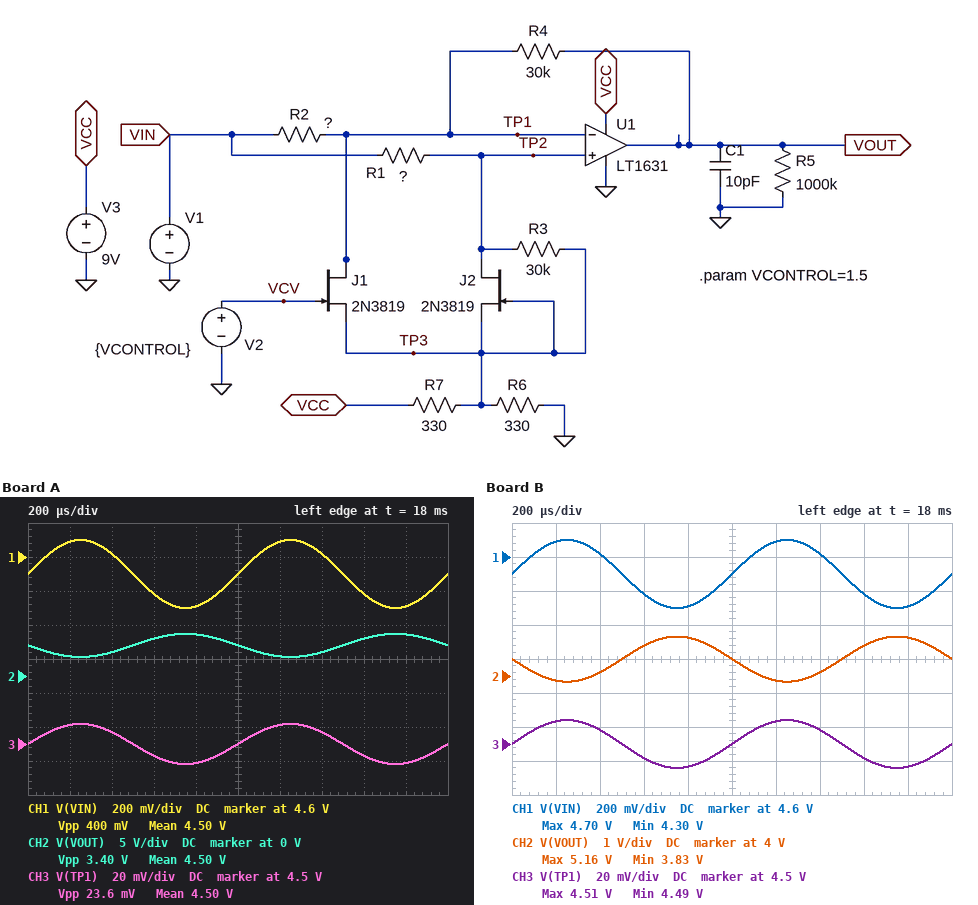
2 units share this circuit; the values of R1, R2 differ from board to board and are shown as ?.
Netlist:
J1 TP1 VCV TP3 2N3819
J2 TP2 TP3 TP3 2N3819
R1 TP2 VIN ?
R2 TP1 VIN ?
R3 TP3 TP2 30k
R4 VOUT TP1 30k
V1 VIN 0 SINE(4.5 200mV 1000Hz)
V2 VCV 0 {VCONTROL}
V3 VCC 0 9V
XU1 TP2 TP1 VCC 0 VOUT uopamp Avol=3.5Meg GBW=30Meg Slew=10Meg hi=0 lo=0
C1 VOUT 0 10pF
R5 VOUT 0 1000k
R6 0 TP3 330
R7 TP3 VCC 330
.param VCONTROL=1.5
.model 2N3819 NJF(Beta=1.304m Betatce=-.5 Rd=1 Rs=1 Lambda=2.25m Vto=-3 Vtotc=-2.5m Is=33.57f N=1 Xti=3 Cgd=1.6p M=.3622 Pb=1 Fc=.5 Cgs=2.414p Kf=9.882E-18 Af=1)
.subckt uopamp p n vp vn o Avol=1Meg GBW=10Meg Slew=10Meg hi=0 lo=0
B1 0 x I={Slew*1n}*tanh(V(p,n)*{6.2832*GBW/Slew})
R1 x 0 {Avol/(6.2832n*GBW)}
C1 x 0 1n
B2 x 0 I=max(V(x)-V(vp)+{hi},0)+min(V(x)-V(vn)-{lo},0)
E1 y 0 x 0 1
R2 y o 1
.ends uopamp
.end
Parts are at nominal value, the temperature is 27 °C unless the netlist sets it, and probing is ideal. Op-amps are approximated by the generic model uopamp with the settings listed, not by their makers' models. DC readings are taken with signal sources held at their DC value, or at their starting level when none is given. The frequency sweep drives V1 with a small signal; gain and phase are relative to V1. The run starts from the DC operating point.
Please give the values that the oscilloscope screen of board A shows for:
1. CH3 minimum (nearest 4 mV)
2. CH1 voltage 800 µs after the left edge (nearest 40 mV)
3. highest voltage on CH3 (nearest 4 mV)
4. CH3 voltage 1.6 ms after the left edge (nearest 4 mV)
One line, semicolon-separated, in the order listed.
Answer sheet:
4.488 V; 4.32 V; 4.512 V; 4.492 V
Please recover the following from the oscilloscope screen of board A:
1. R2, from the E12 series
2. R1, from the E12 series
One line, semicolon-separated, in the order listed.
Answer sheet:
3.3 kΩ; 4.7 kΩ
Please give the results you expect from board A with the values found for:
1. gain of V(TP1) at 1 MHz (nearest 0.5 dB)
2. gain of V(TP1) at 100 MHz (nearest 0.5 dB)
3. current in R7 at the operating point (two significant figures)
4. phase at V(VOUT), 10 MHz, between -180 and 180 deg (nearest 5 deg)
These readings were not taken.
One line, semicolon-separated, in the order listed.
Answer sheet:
-10.5 dB; -6.0 dB; 14 mA; 100 deg
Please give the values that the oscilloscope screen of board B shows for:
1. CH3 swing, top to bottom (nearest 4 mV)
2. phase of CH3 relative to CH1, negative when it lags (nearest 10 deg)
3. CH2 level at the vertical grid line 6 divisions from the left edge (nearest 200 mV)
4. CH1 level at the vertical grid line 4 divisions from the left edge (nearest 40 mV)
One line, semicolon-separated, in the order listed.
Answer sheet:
28 mV; 0 deg; 3.8 V; 4.32 V
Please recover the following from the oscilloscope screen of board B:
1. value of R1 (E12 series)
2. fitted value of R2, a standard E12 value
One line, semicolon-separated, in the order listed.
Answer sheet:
3.9 kΩ; 8.2 kΩ
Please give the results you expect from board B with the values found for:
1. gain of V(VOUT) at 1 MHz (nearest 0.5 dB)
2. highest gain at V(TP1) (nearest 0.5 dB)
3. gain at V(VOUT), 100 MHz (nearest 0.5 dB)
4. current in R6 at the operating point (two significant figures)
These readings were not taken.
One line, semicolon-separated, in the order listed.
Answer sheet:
10.5 dB; -2.0 dB; -23.5 dB; 14 mA
